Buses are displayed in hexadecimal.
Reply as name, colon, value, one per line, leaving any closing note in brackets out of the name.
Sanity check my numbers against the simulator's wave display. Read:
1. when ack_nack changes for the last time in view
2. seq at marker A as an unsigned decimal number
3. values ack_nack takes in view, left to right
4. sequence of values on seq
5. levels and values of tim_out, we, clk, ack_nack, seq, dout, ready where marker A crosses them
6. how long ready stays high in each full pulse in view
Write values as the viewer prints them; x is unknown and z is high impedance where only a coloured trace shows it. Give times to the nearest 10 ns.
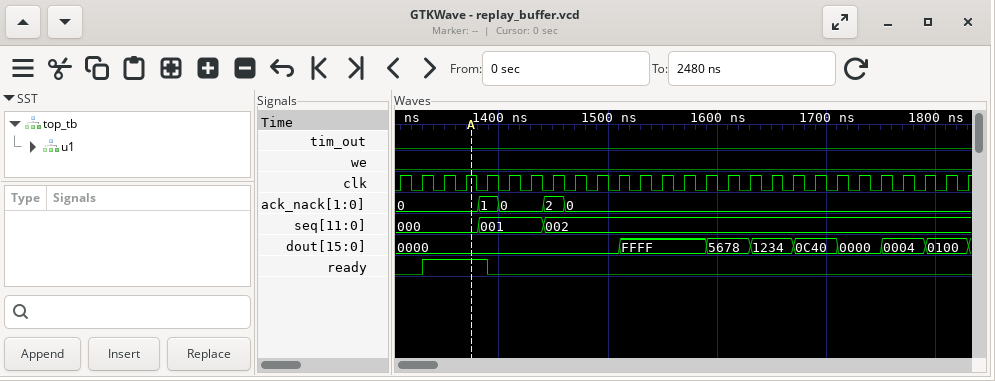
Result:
when ack_nack changes for the last time in view: 1460 ns
seq at marker A as an unsigned decimal number: 0
values ack_nack takes in view, left to right: 0, 1, 0, 2, 0
sequence of values on seq: 000, 001, 002
levels and values of tim_out, we, clk, ack_nack, seq, dout, ready where marker A crosses them: tim_out=0, we=0, clk=1, ack_nack=0, seq=000, dout=0000, ready=1
how long ready stays high in each full pulse in view: 60 ns
